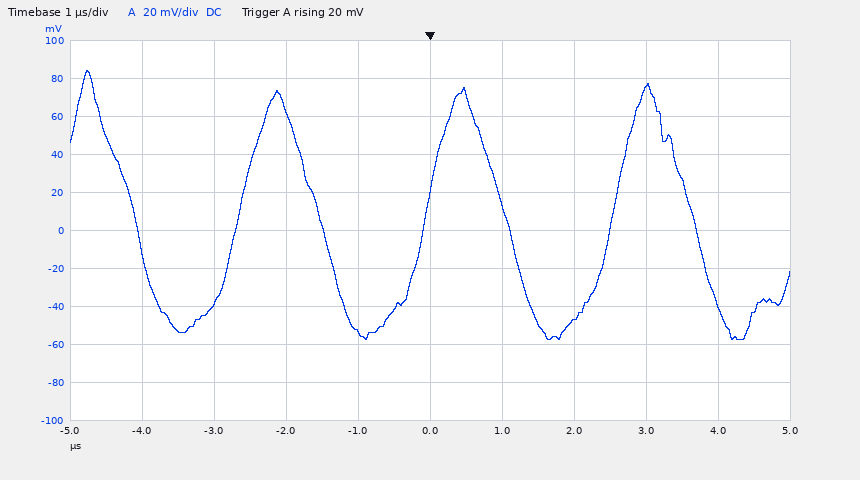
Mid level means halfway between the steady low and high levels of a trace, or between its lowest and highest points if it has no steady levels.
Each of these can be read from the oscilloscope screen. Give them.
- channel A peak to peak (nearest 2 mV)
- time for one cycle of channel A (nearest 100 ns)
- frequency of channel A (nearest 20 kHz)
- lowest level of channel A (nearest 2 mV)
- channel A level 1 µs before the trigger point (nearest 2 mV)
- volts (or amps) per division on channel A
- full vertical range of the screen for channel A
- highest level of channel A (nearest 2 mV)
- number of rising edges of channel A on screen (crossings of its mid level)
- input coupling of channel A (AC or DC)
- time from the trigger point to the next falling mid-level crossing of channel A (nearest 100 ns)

142 mV
2.6 µs
380 kHz
-58 mV
-54 mV
20 mV
200 mV
84 mV
3
DC
1.0 µs
